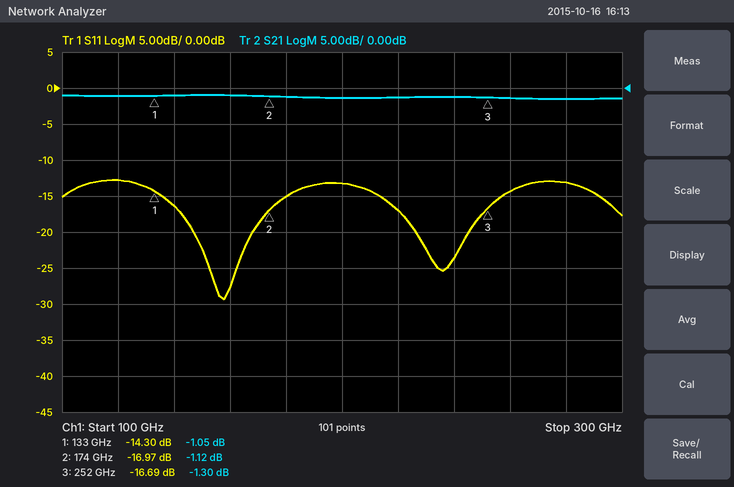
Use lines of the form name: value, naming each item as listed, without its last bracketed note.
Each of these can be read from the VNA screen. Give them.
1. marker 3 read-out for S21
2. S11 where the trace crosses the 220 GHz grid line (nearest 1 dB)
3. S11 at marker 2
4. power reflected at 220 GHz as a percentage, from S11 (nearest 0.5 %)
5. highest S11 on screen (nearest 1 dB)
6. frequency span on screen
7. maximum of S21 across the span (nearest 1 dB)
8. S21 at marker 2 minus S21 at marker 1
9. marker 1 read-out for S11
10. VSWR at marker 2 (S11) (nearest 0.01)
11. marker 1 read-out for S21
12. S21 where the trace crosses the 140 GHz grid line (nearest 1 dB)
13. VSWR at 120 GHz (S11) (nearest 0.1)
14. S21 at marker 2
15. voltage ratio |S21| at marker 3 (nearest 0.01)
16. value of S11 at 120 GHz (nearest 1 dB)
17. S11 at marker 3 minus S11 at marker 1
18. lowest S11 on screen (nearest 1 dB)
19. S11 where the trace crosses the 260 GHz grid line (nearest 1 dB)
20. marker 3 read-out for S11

marker 3 read-out for S21: -1.30 dB
S11 where the trace crosses the 220 GHz grid line: -17 dB
S11 at marker 2: -16.97 dB
power reflected at 220 GHz as a percentage, from S11: 2.0 %
highest S11 on screen: -13 dB
frequency span on screen: 200 GHz
maximum of S21 across the span: -1 dB
S21 at marker 2 minus S21 at marker 1: -0.07 dB
marker 1 read-out for S11: -14.30 dB
VSWR at marker 2 (S11): 1.33
marker 1 read-out for S21: -1.05 dB
S21 where the trace crosses the 140 GHz grid line: -1 dB
VSWR at 120 GHz (S11): 1.6
S21 at marker 2: -1.12 dB
voltage ratio |S21| at marker 3: 0.86
value of S11 at 120 GHz: -13 dB
S11 at marker 3 minus S11 at marker 1: -2.39 dB
lowest S11 on screen: -29 dB
S11 where the trace crosses the 260 GHz grid line: -14 dB
marker 3 read-out for S11: -16.69 dB
